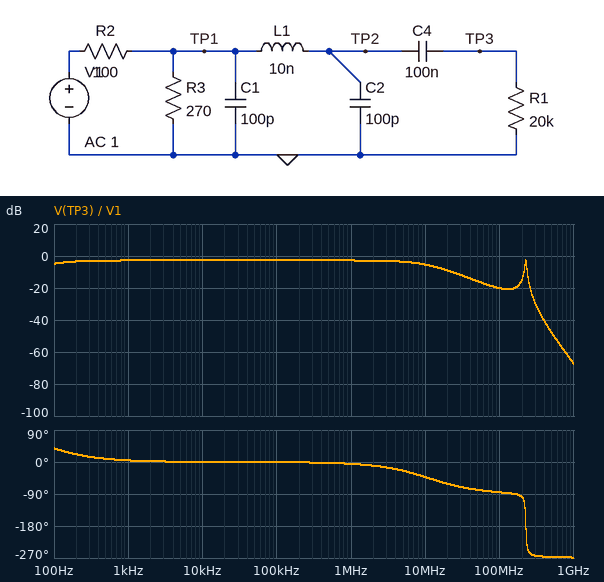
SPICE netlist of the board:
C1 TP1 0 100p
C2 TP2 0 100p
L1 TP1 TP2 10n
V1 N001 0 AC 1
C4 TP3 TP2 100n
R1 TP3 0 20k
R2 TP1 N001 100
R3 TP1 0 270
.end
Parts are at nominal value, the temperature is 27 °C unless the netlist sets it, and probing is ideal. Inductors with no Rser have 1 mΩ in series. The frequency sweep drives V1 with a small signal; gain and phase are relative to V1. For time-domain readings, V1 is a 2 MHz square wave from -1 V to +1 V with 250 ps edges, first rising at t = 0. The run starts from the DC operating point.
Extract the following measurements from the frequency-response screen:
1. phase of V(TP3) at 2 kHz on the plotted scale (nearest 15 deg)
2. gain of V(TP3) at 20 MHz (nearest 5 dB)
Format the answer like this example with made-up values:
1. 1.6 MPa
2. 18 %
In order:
1. 0 deg
2. -10 dB
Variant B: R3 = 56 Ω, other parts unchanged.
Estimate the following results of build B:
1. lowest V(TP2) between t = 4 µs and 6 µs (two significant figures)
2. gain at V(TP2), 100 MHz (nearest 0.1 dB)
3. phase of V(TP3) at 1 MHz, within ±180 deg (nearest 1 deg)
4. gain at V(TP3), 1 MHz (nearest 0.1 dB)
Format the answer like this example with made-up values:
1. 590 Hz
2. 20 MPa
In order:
1. -360 mV
2. -20.2 dB
3. -3 deg
4. -8.9 dB
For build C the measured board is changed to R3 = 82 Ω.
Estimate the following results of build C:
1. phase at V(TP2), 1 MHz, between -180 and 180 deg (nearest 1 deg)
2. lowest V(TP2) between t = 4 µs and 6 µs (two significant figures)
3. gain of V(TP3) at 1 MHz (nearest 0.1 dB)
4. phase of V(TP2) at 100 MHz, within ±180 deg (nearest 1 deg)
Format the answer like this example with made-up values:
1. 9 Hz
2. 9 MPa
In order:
1. -3 deg
2. -450 mV
3. -7.0 dB
4. -82 deg
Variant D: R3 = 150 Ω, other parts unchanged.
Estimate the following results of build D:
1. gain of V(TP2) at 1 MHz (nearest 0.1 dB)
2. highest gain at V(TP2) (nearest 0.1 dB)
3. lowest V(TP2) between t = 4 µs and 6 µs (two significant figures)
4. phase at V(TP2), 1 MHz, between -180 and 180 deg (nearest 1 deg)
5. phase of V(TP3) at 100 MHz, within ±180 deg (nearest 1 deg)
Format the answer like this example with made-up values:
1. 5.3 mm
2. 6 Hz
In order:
1. -4.5 dB
2. -4.4 dB
3. -600 mV
4. -4 deg
5. -84 deg
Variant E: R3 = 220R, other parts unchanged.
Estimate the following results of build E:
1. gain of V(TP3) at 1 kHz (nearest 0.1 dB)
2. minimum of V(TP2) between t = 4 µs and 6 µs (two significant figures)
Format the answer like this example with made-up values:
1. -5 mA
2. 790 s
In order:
1. -3.3 dB
2. -690 mV
